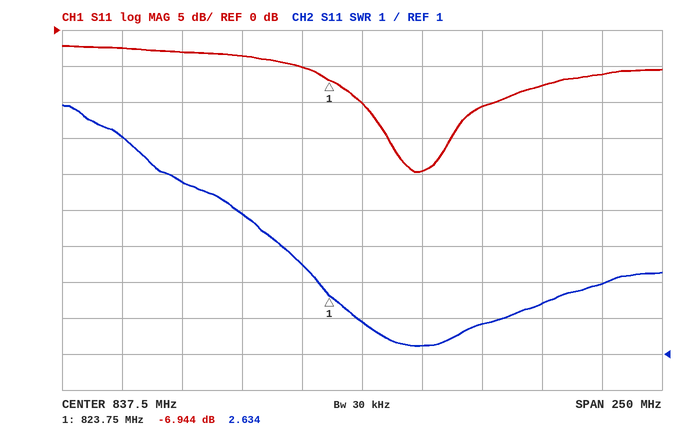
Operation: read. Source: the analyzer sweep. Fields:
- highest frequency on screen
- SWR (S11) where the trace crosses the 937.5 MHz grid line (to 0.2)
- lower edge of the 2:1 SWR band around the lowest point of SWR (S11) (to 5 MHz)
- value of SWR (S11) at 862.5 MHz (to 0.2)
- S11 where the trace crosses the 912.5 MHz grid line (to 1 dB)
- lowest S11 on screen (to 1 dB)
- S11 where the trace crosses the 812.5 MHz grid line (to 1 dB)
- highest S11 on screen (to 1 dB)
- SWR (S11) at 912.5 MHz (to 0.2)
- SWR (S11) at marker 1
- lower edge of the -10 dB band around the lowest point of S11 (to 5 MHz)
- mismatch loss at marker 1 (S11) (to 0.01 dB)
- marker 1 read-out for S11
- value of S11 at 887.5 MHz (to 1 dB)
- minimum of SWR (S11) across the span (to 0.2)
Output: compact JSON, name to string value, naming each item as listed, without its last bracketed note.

{"highest frequency on screen": "962.5 MHz", "SWR (S11) where the trace crosses the 937.5 MHz grid line": "3.0", "lower edge of the 2:1 SWR band around the lowest point of SWR (S11)": "835 MHz", "value of SWR (S11) at 862.5 MHz": "1.2", "S11 where the trace crosses the 912.5 MHz grid line": "-8 dB", "lowest S11 on screen": "-20 dB", "S11 where the trace crosses the 812.5 MHz grid line": "-5 dB", "highest S11 on screen": "-2 dB", "SWR (S11) at 912.5 MHz": "2.4", "SWR (S11) at marker 1": "2.634", "lower edge of the -10 dB band around the lowest point of S11": "835 MHz", "mismatch loss at marker 1 (S11)": "0.98 dB", "marker 1 read-out for S11": "-6.944 dB", "value of S11 at 887.5 MHz": "-11 dB", "minimum of SWR (S11) across the span": "1.2"}
